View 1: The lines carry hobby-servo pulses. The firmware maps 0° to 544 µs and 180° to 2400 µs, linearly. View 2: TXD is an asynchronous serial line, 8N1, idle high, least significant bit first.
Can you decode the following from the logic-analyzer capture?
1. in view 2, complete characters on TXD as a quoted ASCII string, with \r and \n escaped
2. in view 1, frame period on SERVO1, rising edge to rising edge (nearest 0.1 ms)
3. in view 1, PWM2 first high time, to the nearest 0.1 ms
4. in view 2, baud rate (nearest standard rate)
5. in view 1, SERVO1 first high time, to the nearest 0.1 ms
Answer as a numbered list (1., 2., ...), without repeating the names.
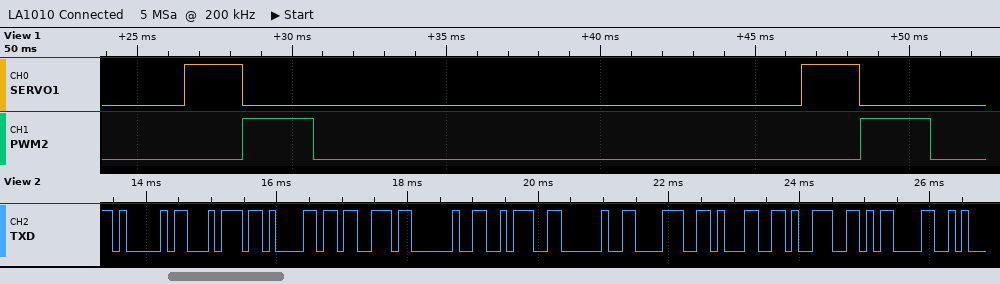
1. "Atas : 819\r"
2. 20.0 ms
3. 2.3 ms
4. 9600 baud
5. 1.9 ms
